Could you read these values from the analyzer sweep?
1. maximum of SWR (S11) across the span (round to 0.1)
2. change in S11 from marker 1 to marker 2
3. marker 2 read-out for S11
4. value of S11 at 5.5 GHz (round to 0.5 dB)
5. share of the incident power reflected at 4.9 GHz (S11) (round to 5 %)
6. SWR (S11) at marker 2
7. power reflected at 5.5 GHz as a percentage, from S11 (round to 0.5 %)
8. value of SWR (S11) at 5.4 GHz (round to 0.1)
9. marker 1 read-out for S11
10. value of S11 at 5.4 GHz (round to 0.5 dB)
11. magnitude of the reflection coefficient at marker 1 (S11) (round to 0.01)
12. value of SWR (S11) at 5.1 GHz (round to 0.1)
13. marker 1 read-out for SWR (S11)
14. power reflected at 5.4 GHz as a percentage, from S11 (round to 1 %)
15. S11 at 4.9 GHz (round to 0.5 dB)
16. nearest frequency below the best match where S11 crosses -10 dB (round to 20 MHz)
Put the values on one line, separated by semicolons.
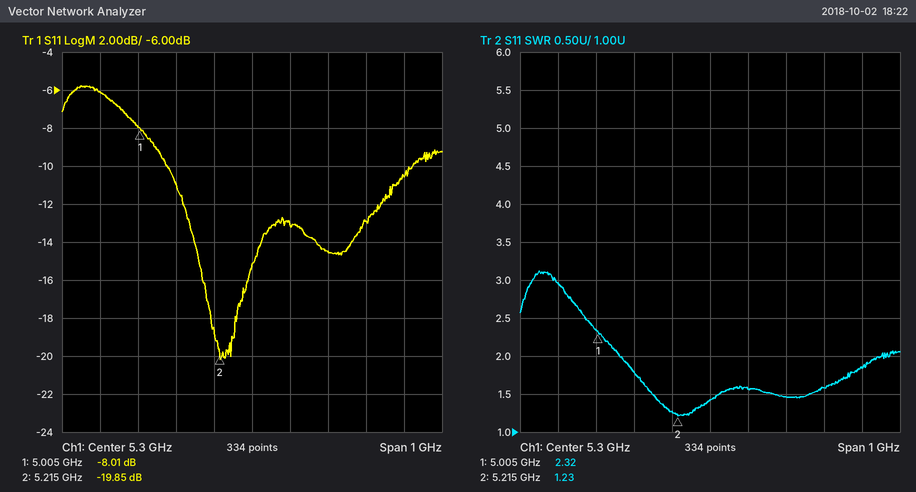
3.1; -11.84 dB; -19.85 dB; -14.5 dB; 25 %; 1.23; 3.5 %; 1.6; -8.01 dB; -13.0 dB; 0.40; 1.8; 2.32; 5 %; -6.0 dB; 5.08 GHz
